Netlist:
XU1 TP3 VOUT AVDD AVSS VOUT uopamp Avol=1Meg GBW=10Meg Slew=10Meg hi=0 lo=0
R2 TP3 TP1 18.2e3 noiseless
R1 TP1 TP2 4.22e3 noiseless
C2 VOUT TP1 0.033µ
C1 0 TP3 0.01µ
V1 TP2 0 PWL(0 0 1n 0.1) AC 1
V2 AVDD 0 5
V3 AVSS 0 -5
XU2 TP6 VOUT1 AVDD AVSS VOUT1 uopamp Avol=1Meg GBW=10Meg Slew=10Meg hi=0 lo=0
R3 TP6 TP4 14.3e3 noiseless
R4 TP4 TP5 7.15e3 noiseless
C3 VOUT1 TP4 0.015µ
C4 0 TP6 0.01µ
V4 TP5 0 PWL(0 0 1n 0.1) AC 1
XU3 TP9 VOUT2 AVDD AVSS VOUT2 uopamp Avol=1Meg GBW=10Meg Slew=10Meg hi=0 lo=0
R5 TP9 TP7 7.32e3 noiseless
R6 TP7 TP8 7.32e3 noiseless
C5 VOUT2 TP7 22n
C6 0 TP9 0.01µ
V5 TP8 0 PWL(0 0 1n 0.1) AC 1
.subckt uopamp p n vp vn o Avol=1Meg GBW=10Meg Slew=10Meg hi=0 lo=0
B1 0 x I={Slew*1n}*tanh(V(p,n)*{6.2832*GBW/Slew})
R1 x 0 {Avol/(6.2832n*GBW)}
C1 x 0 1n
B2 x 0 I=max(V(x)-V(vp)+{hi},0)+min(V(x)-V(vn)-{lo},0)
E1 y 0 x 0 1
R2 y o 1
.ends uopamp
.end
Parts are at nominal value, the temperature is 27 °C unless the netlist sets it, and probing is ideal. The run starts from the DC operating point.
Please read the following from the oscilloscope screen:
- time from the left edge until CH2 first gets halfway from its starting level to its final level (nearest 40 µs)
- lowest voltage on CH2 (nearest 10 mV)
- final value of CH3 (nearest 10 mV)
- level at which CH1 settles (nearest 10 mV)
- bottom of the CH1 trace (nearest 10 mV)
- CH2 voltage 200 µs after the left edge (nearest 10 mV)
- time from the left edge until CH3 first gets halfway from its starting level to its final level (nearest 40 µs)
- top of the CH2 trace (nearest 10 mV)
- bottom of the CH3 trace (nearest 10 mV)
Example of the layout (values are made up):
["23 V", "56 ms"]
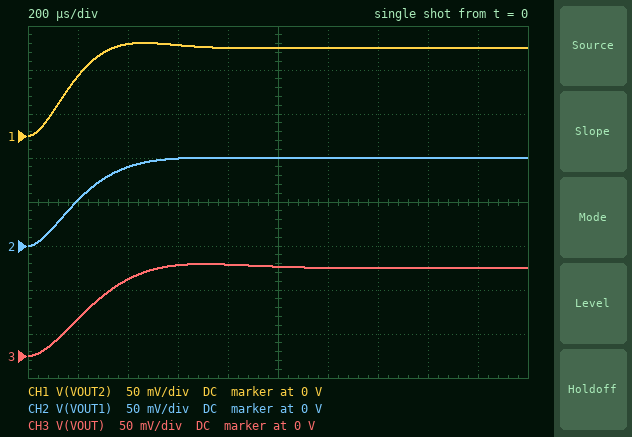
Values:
["200 µs", "0 V", "100 mV", "100 mV", "0 V", "50 mV", "240 µs", "100 mV", "0 V"]
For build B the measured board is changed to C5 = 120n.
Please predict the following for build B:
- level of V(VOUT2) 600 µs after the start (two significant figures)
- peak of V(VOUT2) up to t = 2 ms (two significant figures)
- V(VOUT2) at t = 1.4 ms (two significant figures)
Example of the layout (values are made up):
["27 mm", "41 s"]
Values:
["120 mV", "140 mV", "94 mV"]
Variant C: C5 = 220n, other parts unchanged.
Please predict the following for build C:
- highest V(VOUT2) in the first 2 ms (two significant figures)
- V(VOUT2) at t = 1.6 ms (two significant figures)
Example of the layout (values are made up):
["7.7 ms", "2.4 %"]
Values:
["150 mV", "110 mV"]
